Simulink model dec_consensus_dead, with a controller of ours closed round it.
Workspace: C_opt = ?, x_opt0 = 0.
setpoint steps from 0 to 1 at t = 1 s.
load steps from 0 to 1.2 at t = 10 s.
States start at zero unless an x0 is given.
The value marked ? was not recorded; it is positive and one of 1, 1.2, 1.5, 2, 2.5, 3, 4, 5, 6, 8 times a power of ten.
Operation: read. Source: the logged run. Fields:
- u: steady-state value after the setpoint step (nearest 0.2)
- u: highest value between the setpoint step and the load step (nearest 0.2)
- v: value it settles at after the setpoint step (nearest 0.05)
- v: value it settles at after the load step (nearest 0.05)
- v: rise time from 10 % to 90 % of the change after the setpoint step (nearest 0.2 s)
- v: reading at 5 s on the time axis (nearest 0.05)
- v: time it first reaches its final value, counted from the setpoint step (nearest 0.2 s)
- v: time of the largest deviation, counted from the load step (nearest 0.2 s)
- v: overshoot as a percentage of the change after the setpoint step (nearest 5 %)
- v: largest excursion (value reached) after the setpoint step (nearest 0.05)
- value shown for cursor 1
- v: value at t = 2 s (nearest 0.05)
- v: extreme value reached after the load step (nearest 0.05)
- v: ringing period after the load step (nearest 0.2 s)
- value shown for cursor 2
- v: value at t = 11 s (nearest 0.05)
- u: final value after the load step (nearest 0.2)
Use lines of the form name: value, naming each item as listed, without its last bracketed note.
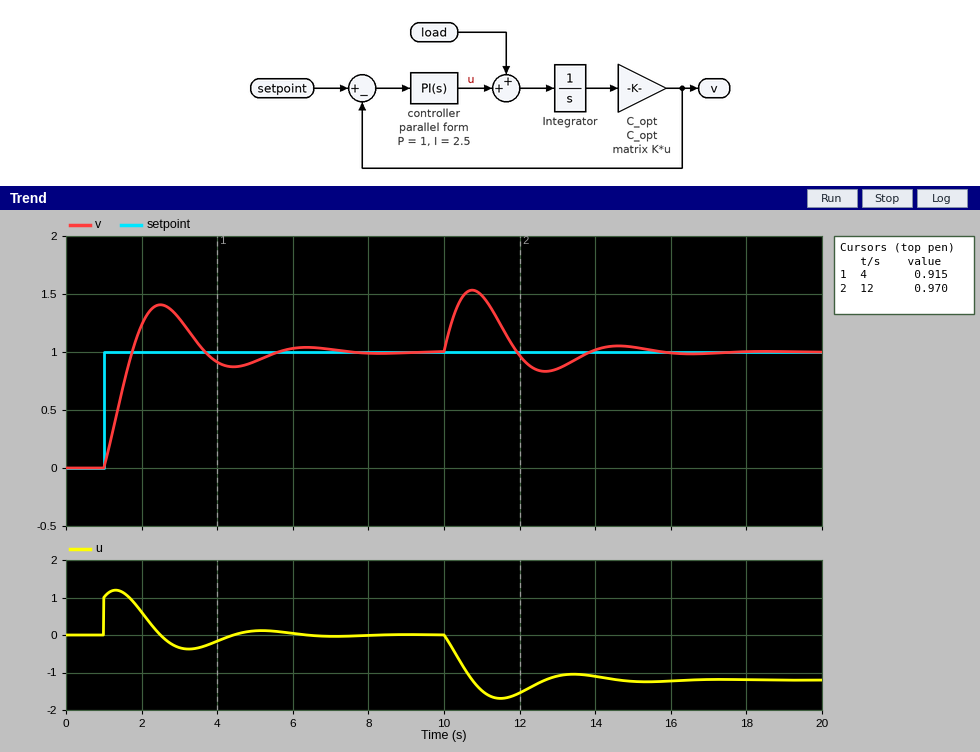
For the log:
u: steady-state value after the setpoint step: 0.0
u: highest value between the setpoint step and the load step: 1.2
v: value it settles at after the setpoint step: 1.00
v: value it settles at after the load step: 1.00
v: rise time from 10 % to 90 % of the change after the setpoint step: 0.6 s
v: reading at 5 s on the time axis: 0.90
v: time it first reaches its final value, counted from the setpoint step: 0.8 s
v: time of the largest deviation, counted from the load step: 0.8 s
v: overshoot as a percentage of the change after the setpoint step: 40 %
v: largest excursion (value reached) after the setpoint step: 1.40
value shown for cursor 1: 0.915
v: value at t = 2 s: 1.25
v: extreme value reached after the load step: 1.55
v: ringing period after the load step: 3.8 s
value shown for cursor 2: 0.970
v: value at t = 11 s: 1.50
u: final value after the load step: -1.2
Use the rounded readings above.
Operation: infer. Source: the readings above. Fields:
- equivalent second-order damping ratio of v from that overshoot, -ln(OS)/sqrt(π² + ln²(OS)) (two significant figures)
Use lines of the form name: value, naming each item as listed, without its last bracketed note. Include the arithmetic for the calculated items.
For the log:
equivalent second-order damping ratio of v from that overshoot, -ln(OS)/sqrt(π² + ln²(OS)): ln(0.4) = -0.916; 0.916 / sqrt(9.870 + 0.840) = 0.28
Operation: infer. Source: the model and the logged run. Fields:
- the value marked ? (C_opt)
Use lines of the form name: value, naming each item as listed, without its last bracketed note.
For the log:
the value marked ?: 1.2
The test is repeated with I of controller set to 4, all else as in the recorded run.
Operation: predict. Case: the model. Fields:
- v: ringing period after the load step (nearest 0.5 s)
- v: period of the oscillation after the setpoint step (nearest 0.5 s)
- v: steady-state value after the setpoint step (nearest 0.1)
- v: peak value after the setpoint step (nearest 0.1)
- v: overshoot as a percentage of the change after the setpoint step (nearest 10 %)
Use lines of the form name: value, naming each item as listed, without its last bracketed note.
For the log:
v: ringing period after the load step: 3.0 s
v: period of the oscillation after the setpoint step: 3.0 s
v: steady-state value after the setpoint step: 1.0
v: peak value after the setpoint step: 1.5
v: overshoot as a percentage of the change after the setpoint step: 50 %
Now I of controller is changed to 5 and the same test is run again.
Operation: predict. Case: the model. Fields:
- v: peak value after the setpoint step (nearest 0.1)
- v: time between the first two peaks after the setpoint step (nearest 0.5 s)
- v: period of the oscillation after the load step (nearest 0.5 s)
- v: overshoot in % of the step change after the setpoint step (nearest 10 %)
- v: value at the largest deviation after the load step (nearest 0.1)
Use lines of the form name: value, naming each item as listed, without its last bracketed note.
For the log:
v: peak value after the setpoint step: 1.5
v: time between the first two peaks after the setpoint step: 2.5 s
v: period of the oscillation after the load step: 2.5 s
v: overshoot in % of the step change after the setpoint step: 50 %
v: value at the largest deviation after the load step: 1.4
